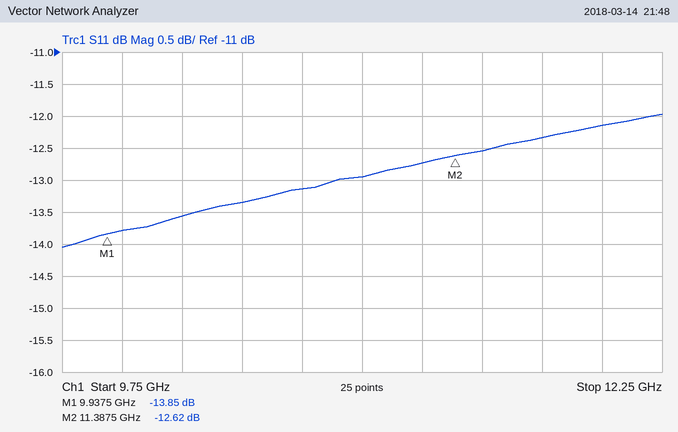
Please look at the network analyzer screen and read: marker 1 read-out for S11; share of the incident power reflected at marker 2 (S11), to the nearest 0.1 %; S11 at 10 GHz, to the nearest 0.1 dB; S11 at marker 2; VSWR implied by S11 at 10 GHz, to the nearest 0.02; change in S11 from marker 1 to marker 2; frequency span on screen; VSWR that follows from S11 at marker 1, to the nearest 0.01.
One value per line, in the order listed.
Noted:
-13.85 dB
5.5 %
-13.8 dB
-12.62 dB
1.52
1.23 dB
2.5 GHz
1.51
